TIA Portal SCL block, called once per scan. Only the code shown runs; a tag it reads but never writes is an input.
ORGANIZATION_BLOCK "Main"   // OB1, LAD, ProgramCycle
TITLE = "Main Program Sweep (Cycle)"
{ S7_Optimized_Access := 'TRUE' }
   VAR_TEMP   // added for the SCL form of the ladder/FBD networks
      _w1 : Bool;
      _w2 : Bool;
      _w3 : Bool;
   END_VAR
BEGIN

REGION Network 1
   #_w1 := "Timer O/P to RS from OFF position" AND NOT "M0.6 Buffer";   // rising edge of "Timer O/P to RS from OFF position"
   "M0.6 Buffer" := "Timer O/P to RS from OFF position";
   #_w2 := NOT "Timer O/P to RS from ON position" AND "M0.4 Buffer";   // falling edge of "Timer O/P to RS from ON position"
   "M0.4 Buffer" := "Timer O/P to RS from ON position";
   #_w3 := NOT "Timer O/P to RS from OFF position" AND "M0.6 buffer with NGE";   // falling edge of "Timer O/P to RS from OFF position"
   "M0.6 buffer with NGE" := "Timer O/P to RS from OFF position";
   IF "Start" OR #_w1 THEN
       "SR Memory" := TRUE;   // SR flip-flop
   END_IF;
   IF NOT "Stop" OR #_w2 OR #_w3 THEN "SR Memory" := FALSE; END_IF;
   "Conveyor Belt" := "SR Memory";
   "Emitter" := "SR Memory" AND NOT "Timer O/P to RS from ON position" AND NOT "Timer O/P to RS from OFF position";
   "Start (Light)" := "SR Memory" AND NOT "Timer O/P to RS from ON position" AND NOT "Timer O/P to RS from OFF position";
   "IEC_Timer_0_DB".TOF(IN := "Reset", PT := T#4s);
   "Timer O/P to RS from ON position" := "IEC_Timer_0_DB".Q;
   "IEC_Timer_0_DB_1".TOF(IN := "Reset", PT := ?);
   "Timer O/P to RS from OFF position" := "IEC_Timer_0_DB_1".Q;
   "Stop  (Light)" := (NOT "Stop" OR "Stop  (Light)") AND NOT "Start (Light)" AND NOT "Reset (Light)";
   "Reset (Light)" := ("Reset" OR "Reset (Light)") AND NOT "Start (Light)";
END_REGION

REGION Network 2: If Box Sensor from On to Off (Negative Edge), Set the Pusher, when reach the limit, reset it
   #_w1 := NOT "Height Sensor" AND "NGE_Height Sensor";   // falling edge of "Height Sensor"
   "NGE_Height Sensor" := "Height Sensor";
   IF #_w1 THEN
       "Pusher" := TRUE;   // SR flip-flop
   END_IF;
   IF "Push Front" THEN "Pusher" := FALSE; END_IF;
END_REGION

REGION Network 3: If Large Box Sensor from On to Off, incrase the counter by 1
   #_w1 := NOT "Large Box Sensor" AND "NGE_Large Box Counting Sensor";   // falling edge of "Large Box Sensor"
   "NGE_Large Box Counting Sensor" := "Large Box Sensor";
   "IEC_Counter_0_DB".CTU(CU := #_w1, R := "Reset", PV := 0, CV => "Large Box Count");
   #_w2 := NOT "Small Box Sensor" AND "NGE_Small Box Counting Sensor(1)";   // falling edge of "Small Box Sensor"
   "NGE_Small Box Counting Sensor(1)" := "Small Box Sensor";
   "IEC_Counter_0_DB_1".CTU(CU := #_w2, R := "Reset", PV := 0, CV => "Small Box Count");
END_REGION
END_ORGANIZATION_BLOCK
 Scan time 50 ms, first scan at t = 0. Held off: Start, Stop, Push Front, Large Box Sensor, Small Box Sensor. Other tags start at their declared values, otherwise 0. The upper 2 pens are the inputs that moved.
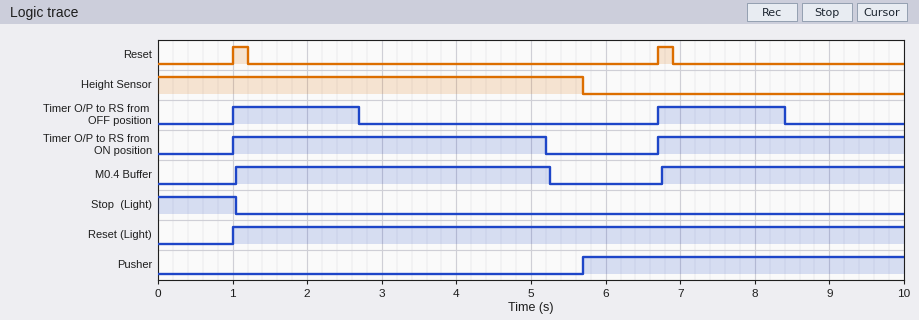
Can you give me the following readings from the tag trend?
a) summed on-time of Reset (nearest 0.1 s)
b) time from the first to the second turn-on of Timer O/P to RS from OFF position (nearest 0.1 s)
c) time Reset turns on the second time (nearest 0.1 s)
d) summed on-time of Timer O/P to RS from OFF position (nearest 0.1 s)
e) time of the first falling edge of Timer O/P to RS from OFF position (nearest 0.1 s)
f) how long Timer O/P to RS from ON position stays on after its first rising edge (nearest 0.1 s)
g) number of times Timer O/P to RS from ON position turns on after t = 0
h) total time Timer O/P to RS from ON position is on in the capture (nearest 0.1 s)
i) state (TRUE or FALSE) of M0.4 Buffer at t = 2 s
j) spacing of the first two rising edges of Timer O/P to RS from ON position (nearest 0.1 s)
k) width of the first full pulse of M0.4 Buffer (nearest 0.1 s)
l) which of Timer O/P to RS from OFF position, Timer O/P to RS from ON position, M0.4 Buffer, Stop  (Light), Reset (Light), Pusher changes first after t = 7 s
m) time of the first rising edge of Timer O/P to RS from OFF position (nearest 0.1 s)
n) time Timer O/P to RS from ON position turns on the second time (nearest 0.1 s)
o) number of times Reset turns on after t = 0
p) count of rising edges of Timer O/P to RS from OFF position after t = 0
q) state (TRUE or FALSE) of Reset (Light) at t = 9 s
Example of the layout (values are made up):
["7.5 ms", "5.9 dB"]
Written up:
["0.4 s", "5.7 s", "6.7 s", "3.4 s", "2.7 s", "4.2 s", "2", "7.5 s", "TRUE", "5.7 s", "4.2 s", "Timer O/P to RS from OFF position", "1.0 s", "6.7 s", "2", "2", "TRUE"]
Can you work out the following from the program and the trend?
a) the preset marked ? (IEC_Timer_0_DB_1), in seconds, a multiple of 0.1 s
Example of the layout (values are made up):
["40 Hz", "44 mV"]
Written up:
["1.5 s"]
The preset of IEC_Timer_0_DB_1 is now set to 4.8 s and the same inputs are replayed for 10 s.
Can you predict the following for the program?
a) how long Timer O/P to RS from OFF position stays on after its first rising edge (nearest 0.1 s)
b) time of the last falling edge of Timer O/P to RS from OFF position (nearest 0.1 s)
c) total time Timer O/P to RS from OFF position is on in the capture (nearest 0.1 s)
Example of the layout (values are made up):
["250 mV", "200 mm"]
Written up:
["5.0 s", "6.0 s", "8.3 s"]
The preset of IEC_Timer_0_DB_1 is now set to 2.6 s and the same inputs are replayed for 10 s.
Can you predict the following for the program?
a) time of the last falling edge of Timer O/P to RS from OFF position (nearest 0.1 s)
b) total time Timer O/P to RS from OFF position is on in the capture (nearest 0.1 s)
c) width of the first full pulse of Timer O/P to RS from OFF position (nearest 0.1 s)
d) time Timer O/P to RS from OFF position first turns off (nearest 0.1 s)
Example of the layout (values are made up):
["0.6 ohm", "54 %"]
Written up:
["9.5 s", "5.6 s", "2.8 s", "3.8 s"]
